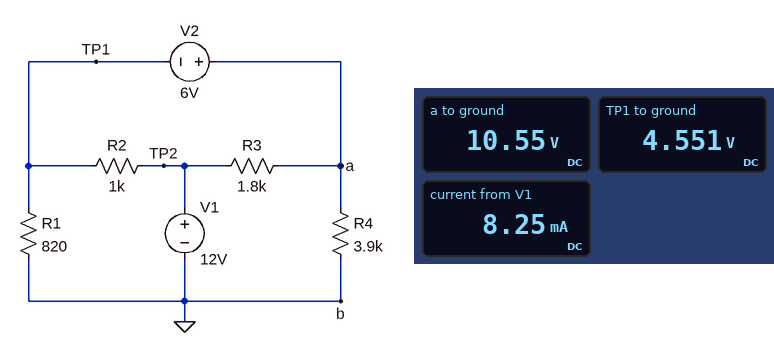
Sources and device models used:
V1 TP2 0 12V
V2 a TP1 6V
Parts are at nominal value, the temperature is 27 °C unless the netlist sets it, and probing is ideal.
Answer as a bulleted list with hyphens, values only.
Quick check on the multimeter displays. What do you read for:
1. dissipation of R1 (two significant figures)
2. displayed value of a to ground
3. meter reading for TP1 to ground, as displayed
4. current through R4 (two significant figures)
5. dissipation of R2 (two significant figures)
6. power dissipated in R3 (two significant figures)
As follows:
- 25 mW
- 10.55 V
- 4.551 V
- 2.7 mA
- 55 mW
- 1.2 mW
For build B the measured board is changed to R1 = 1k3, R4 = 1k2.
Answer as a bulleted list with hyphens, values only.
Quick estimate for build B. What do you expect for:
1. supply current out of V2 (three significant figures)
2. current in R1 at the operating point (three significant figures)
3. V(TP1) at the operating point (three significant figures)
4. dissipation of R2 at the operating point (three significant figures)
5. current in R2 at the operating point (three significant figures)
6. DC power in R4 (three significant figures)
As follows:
- 6.21 mA
- 2.52 mA
- 3.27 V
- 76.2 mW
- 8.73 mA
- 71.6 mW
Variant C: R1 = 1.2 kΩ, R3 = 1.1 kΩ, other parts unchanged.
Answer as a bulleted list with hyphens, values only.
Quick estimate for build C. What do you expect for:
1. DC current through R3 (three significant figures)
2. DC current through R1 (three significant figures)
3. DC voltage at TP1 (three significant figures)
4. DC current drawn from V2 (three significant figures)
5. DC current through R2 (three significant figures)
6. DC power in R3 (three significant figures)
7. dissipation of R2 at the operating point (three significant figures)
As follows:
- 630 µA
- 4.42 mA
- 5.31 V
- 2.27 mA
- 6.69 mA
- 436 µW
- 44.8 mW
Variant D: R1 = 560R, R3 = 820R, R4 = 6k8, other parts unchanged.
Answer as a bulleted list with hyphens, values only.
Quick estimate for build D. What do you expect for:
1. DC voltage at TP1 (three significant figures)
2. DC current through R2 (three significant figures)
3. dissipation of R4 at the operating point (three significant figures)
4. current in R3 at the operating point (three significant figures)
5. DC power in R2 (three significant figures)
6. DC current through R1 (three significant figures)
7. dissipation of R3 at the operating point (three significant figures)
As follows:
- 4.44 V
- 7.56 mA
- 16.0 mW
- 1.90 mA
- 57.2 mW
- 7.93 mA
- 2.97 mW
